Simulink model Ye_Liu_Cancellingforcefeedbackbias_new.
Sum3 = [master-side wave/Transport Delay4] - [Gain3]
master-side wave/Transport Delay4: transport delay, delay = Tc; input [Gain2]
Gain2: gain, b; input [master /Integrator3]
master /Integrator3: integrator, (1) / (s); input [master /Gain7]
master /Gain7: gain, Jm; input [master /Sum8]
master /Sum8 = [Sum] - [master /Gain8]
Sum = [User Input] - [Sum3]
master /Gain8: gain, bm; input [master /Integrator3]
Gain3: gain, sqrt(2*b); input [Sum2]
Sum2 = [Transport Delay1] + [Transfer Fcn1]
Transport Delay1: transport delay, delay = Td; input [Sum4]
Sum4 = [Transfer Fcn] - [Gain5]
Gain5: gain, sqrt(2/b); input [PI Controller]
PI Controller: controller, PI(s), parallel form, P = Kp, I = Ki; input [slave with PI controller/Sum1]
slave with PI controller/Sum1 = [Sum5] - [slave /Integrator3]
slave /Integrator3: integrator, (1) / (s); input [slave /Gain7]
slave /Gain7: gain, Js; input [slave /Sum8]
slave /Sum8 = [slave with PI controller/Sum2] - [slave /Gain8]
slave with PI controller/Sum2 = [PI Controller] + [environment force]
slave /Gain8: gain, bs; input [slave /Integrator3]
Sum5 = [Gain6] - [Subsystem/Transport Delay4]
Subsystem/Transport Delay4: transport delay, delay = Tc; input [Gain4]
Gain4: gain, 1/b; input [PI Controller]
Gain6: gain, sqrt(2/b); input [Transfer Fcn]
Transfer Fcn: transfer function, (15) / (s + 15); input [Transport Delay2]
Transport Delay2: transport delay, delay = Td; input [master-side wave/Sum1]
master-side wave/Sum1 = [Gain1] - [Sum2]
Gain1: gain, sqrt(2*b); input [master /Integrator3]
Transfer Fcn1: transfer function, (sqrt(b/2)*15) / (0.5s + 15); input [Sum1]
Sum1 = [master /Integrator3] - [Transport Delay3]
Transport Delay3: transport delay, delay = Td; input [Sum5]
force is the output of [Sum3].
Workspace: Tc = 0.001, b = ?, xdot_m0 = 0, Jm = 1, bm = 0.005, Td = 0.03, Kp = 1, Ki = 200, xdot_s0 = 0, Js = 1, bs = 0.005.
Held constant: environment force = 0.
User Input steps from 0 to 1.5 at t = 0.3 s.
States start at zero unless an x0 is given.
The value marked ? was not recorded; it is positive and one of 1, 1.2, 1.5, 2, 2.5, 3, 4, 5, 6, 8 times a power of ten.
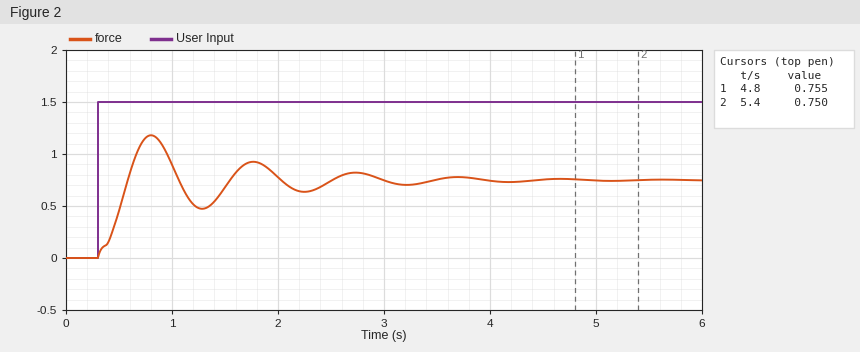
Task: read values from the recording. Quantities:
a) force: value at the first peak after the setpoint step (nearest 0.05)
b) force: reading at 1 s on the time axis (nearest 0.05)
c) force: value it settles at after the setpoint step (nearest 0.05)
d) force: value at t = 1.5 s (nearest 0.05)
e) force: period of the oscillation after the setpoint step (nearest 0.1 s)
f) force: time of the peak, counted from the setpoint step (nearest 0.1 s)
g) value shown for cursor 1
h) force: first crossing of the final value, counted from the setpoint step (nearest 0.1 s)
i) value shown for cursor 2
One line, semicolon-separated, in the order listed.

1.20; 0.90; 0.75; 0.70; 1.0 s; 0.5 s; 0.755; 0.3 s; 0.750
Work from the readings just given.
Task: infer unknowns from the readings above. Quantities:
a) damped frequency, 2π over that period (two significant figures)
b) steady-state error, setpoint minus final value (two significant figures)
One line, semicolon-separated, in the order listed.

6.3 rad/s; 0.75
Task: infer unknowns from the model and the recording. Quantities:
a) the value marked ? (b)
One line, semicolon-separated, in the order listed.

3
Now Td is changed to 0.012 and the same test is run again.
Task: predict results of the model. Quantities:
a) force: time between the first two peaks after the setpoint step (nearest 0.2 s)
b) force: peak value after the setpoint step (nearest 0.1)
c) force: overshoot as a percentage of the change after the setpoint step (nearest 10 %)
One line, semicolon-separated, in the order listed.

0.8 s; 1.1; 50 %
